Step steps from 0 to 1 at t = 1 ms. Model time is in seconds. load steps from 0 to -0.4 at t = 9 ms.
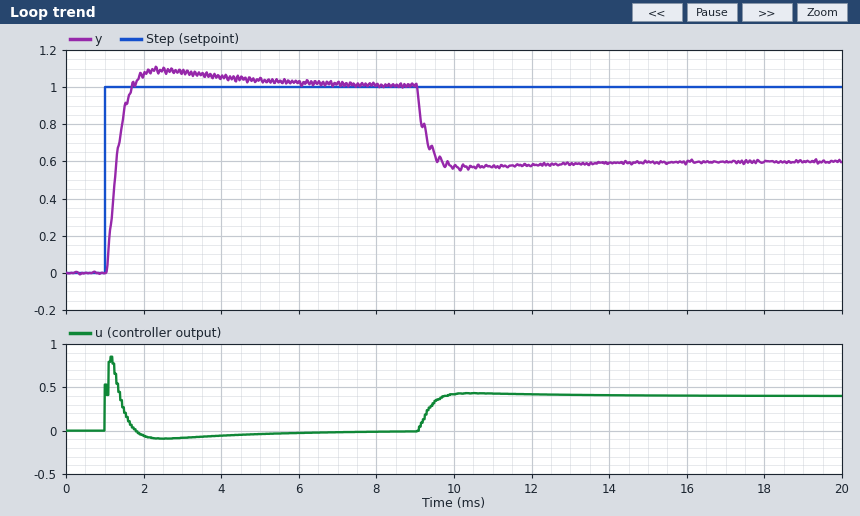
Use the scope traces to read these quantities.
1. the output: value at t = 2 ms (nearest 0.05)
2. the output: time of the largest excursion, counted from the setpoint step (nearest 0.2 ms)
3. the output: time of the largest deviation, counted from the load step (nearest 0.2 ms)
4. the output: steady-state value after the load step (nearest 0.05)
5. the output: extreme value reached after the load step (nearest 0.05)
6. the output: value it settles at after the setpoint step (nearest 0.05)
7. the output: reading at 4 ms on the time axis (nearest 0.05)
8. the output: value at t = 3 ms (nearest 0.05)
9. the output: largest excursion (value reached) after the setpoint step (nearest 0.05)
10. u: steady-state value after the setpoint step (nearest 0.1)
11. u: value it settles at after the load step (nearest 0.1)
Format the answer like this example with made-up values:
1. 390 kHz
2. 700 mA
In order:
1. 1.05
2. 1.4 ms
3. 1.2 ms
4. 0.60
5. 0.55
6. 1.00
7. 1.05
8. 1.10
9. 1.10
10. 0.0
11. 0.4
